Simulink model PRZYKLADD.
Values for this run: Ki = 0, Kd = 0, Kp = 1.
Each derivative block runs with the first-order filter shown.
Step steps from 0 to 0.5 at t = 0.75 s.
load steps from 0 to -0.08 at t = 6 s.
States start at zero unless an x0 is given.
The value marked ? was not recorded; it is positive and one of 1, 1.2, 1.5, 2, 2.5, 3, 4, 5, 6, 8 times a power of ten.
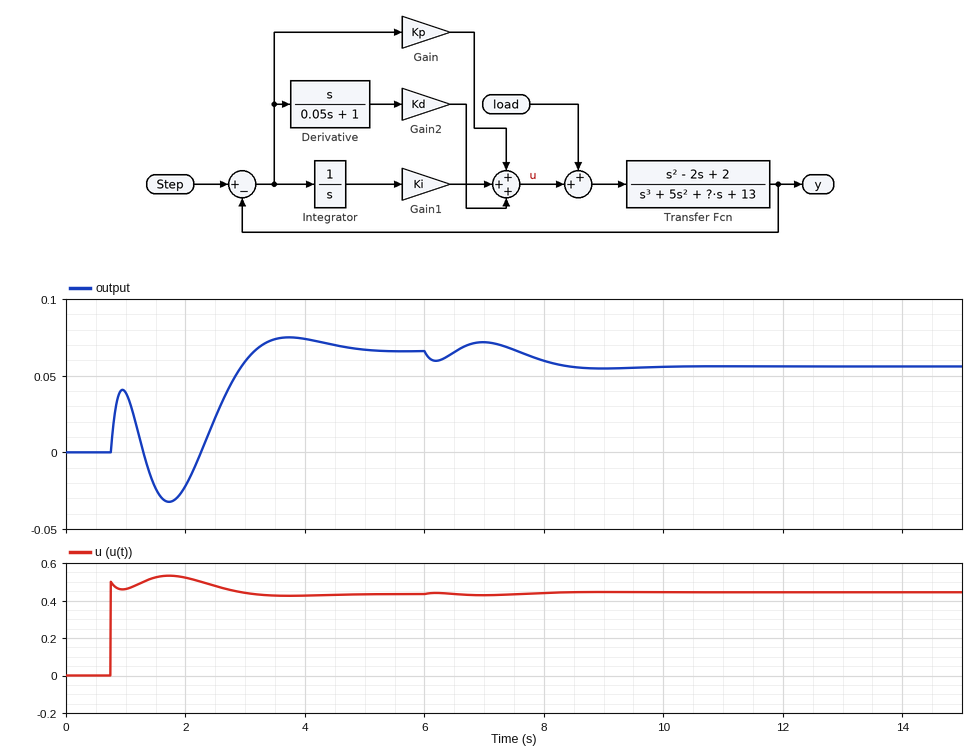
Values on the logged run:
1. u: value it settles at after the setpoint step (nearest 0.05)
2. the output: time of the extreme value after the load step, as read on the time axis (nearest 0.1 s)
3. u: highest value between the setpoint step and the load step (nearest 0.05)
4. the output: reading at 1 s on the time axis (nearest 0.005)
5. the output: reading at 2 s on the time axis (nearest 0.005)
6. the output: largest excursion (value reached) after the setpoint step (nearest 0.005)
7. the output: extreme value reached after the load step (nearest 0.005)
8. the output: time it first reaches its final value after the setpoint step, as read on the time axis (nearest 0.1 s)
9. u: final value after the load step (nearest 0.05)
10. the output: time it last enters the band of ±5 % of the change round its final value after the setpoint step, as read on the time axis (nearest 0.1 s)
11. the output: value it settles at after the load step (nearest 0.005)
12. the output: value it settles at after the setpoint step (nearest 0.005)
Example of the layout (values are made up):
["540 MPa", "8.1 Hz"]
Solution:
["0.45", "9.0 s", "0.55", "0.040", "-0.020", "0.075", "0.055", "3.2 s", "0.45", "4.5 s", "0.055", "0.065"]
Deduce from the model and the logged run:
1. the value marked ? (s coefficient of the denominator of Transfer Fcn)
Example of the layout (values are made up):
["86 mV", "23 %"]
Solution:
["15"]
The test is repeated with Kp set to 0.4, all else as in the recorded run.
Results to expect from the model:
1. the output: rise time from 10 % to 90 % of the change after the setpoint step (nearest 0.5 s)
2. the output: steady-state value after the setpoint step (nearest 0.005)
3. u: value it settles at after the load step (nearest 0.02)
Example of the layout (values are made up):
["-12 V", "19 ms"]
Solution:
["2.5 s", "0.030", "0.20"]
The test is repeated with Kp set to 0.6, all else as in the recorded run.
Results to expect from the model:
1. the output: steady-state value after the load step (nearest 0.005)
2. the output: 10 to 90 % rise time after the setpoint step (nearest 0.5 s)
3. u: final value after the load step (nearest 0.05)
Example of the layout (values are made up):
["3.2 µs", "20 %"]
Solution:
["0.030", "2.5 s", "0.30"]
